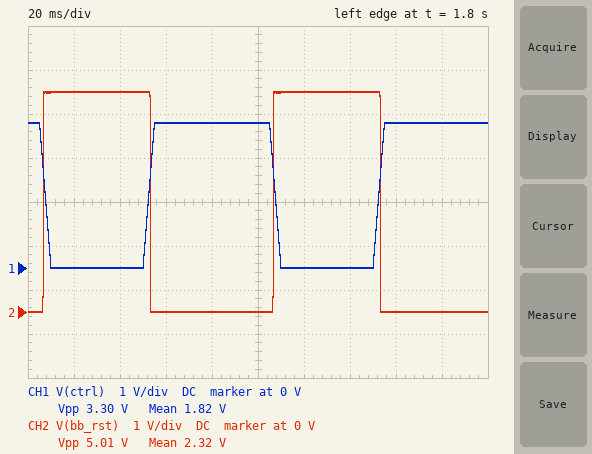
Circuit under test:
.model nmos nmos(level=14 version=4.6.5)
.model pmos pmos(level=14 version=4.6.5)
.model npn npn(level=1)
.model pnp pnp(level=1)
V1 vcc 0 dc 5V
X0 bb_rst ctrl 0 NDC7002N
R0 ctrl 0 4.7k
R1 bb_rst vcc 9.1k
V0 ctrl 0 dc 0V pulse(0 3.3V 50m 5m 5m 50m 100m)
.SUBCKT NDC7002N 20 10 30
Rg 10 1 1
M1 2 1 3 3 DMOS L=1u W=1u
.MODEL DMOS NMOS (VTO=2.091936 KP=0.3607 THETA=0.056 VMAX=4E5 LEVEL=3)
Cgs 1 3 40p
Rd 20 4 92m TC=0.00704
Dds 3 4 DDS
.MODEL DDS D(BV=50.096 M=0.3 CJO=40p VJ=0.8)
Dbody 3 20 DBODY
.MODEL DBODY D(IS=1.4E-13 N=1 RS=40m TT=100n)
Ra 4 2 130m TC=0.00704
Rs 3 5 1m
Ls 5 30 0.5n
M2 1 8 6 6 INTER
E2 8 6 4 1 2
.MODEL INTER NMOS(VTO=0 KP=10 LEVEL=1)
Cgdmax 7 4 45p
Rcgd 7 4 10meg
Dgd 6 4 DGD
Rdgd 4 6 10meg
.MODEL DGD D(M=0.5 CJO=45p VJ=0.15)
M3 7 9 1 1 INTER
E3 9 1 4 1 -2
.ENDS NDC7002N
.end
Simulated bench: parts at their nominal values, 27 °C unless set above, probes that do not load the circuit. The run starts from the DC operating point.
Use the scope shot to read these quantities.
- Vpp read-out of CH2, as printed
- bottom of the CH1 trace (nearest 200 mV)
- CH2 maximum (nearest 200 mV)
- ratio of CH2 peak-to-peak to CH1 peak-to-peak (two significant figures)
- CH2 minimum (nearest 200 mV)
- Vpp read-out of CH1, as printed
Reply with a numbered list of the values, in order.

1. 5.01 V
2. 0 V
3. 5.0 V
4. 1.5
5. 0 V
6. 3.30 V
